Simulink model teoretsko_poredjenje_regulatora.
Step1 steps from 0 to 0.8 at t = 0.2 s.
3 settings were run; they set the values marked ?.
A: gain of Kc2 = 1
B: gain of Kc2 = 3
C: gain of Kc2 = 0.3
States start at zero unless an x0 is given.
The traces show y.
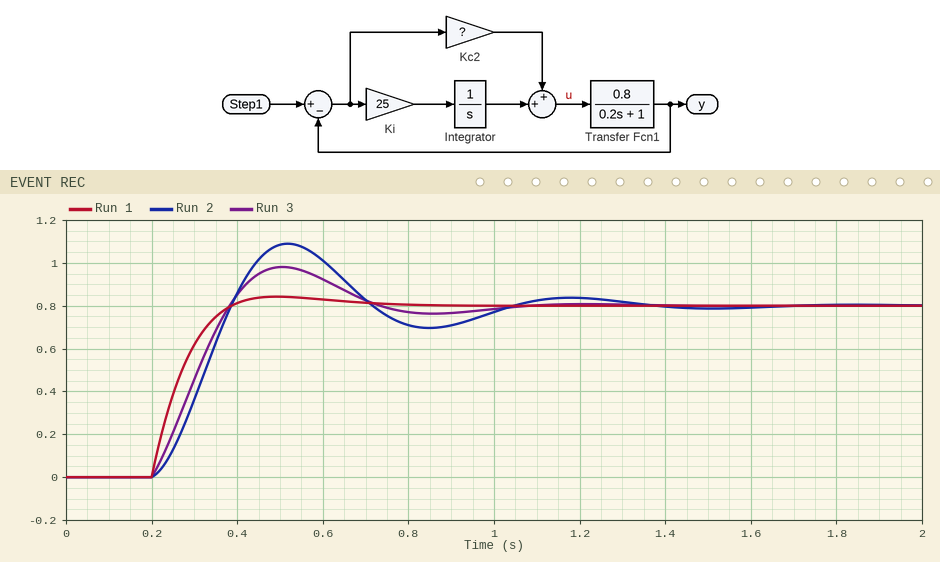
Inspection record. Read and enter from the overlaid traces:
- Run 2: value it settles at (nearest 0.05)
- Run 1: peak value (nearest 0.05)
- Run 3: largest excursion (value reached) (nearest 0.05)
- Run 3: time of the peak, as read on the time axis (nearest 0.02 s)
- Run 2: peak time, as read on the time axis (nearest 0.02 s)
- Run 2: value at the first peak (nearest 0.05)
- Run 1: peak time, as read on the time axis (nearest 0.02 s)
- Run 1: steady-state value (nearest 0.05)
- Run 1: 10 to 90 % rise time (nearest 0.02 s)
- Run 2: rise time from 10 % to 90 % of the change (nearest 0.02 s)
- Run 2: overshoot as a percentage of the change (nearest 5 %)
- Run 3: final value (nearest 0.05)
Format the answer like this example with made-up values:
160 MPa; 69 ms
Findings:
0.80; 0.85; 1.00; 0.50 s; 0.52 s; 1.10; 0.50 s; 0.80; 0.12 s; 0.14 s; 35 %; 0.80
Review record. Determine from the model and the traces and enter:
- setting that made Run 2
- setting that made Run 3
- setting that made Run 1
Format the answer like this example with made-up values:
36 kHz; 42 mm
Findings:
C; A; B
